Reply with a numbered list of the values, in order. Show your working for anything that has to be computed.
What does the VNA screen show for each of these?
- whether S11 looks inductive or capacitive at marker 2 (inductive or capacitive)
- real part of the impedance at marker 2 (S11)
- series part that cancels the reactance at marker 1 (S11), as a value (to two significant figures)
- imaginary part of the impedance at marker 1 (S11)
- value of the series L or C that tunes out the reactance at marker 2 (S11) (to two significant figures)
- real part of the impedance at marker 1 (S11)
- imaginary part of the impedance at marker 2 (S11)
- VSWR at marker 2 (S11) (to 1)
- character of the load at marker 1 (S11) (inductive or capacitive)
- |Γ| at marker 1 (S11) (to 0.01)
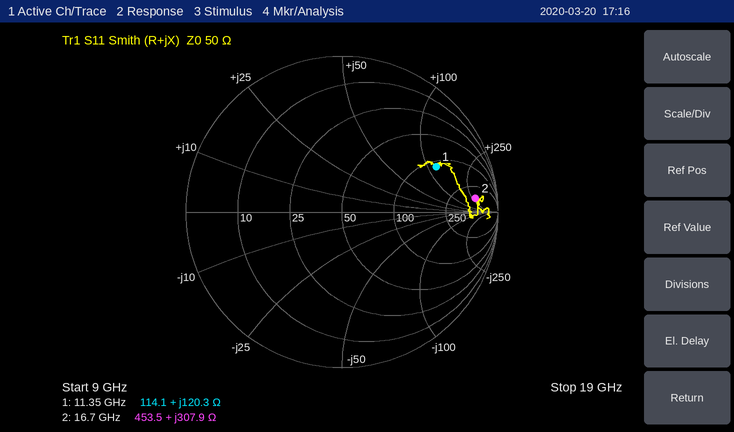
1. inductive
2. 453.5 Ω
3. C = 1/(2π × 11.35 GHz × 120.3 Ω) ≈ 117 fF, so 120 fF to two significant figures
4. +120.3 Ω
5. C = 1/(2π × 16.7 GHz × 307.9 Ω) ≈ 31 fF
6. 114.1 Ω
7. +307.9 Ω
8. 13
9. inductive
10. 0.67
